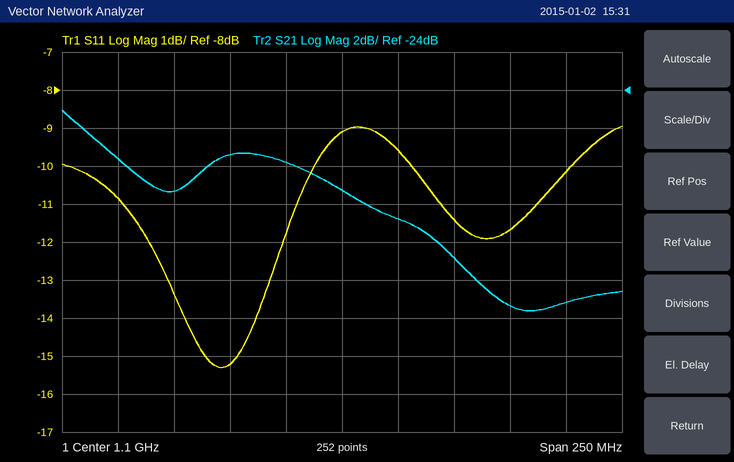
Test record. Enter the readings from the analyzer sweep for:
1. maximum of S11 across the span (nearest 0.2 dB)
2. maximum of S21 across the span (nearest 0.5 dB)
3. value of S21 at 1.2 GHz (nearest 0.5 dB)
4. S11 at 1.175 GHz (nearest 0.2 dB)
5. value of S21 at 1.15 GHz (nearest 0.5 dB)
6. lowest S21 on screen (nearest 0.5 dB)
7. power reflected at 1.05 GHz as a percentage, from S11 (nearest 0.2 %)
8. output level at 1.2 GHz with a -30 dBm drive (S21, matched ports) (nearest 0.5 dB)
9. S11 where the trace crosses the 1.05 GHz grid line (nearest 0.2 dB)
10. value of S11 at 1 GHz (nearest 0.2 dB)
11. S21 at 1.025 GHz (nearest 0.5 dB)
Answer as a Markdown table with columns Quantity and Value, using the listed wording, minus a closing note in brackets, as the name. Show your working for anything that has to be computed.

| Quantity | Value |
|---|---|
| maximum of S11 across the span | -9.0 dB |
| maximum of S21 across the span | -25.0 dB |
| value of S21 at 1.2 GHz | -35.0 dB |
| S11 at 1.175 GHz | -11.6 dB |
| value of S21 at 1.15 GHz | -33.0 dB |
| lowest S21 on screen | -35.5 dB |
| power reflected at 1.05 GHz as a percentage, from S11 | 10^(-15.2/10) ≈ 3.0 % |
| output level at 1.2 GHz with a -30 dBm drive (S21, matched ports) | -30 dBm + (-35.0 dB) = -65.0 dBm |
| S11 where the trace crosses the 1.05 GHz grid line | -15.2 dB |
| value of S11 at 1 GHz | -10.8 dB |
| S21 at 1.025 GHz | -29.5 dB |
